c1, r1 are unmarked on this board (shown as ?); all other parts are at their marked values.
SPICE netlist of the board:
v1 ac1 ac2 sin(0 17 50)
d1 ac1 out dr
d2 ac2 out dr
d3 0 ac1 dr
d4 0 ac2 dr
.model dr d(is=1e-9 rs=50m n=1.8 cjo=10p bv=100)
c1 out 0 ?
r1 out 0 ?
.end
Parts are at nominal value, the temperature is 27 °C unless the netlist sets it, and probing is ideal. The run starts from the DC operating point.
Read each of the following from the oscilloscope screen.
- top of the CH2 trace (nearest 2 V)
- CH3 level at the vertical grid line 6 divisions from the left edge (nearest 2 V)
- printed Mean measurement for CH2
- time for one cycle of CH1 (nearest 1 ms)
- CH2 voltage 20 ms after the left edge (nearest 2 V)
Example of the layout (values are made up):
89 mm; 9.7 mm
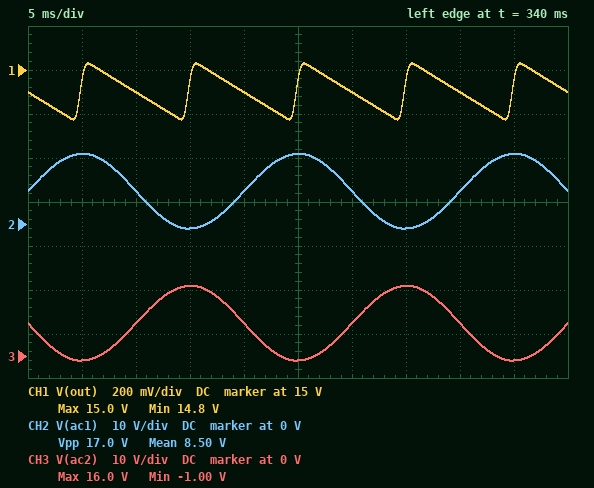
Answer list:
16 V; 8 V; 8.50 V; 10 ms; 8 V
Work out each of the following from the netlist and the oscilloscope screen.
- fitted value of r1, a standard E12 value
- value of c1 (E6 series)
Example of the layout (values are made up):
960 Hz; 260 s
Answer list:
150 Ω; 3.3 mF
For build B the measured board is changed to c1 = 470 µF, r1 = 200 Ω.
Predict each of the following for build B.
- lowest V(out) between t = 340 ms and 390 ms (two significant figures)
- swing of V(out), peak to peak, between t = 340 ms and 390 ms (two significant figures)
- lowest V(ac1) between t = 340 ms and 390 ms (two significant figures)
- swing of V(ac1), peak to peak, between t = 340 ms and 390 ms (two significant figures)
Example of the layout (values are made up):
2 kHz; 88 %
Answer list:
14 V; 1.3 V; -990 mV; 17 V
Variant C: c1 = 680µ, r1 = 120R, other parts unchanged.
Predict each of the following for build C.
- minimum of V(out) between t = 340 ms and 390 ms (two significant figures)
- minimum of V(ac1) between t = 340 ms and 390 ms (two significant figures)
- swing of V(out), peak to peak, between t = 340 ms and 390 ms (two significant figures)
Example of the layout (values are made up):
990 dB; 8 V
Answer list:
14 V; -1.0 V; 1.4 V
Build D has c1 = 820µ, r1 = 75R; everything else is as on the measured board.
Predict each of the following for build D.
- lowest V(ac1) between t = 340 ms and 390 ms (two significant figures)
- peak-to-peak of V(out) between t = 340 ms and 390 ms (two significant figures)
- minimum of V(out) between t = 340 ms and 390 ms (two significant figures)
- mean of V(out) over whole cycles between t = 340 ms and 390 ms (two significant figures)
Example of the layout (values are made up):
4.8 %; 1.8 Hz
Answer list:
-1.1 V; 1.8 V; 13 V; 14 V
